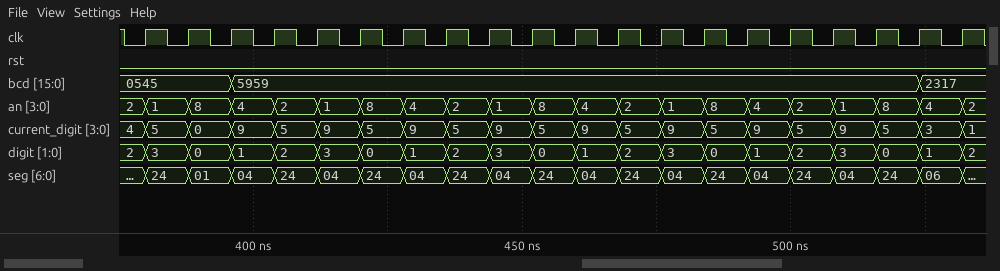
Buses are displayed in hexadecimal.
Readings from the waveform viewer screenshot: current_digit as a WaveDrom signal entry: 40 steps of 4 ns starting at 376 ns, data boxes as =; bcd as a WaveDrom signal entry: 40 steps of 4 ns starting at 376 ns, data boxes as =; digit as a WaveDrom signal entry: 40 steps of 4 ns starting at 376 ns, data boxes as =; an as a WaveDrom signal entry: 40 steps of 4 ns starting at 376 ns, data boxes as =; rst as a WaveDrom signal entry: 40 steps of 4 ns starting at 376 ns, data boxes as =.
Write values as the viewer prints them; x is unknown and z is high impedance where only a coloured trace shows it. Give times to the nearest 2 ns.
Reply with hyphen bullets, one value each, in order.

- {name: 'current_digit', wave: '==.=.=.=.=.=.=.=.=.=.=.=.=.=.=.=.=.=.=.=', data: '4 5 0 9 5 9 5 9 5 9 5 9 5 9 5 9 5 9 5 3 1'}
- {name: 'bcd', wave: '=....=...............................=..', data: '0545 5959 2317'}
- {name: 'digit', wave: '==.=.=.=.=.=.=.=.=.=.=.=.=.=.=.=.=.=.=.=', data: '2 3 0 1 2 3 0 1 2 3 0 1 2 3 0 1 2 3 0 1 2'}
- {name: 'an', wave: '==.=.=.=.=.=.=.=.=.=.=.=.=.=.=.=.=.=.=.=', data: '2 1 8 4 2 1 8 4 2 1 8 4 2 1 8 4 2 1 8 4 2'}
- {name: 'rst', wave: '0.......................................'}
